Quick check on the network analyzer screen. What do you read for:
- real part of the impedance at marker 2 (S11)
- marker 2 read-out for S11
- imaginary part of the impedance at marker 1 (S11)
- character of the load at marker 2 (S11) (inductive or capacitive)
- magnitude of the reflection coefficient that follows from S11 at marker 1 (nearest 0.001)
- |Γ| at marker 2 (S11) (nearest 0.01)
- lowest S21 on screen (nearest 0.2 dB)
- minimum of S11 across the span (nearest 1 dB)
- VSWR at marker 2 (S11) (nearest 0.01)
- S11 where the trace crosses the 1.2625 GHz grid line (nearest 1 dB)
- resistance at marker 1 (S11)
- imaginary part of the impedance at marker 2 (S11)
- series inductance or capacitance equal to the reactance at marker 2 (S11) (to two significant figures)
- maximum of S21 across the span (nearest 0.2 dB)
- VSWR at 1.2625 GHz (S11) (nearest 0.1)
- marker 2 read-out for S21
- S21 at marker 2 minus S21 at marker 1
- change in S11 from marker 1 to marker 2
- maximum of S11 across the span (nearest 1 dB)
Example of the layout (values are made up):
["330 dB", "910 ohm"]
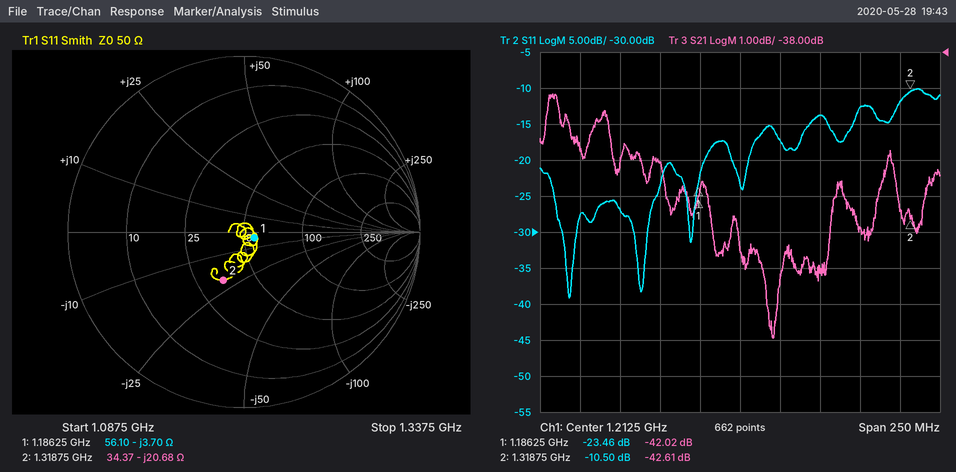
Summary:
["34.37 Ω", "-10.50 dB", "-3.70 Ω", "capacitive", "0.067", "0.30", "-46.0 dB", "-39 dB", "1.85", "-14 dB", "56.10 Ω", "-20.68 Ω", "5.8 pF", "-39.2 dB", "1.5", "-42.61 dB", "-0.59 dB", "12.96 dB", "-10 dB"]
